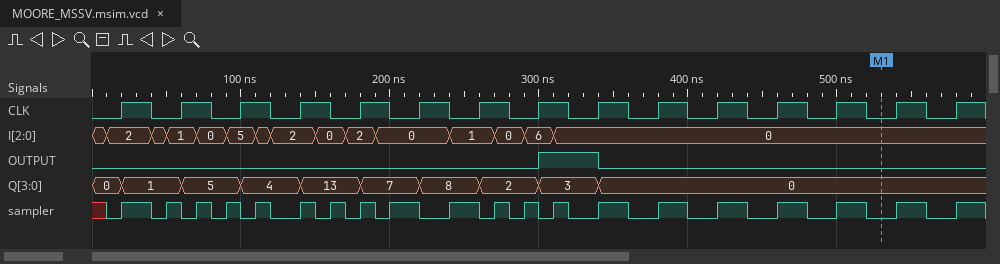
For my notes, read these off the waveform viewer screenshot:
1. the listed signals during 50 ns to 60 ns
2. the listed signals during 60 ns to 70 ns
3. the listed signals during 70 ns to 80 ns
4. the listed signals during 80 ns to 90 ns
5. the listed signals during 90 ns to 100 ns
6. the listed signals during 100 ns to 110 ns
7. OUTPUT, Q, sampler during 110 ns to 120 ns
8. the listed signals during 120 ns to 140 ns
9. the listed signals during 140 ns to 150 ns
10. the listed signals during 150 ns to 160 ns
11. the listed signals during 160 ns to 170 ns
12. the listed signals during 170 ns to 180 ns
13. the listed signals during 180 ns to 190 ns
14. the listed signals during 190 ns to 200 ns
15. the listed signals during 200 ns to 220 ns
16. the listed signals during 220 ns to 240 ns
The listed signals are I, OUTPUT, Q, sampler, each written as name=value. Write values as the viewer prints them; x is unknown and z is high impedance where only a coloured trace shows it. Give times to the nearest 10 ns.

I=1, OUTPUT=0, Q=1, sampler=1
I=1, OUTPUT=0, Q=5, sampler=0
I=0, OUTPUT=0, Q=5, sampler=1
I=0, OUTPUT=0, Q=5, sampler=0
I=5, OUTPUT=0, Q=5, sampler=1
I=5, OUTPUT=0, Q=4, sampler=0
OUTPUT=0, Q=4, sampler=1
I=2, OUTPUT=0, Q=4, sampler=0
I=2, OUTPUT=0, Q=13, sampler=1
I=0, OUTPUT=0, Q=13, sampler=0
I=0, OUTPUT=0, Q=13, sampler=1
I=2, OUTPUT=0, Q=13, sampler=0
I=2, OUTPUT=0, Q=7, sampler=1
I=0, OUTPUT=0, Q=7, sampler=0
I=0, OUTPUT=0, Q=7, sampler=1
I=0, OUTPUT=0, Q=8, sampler=0
